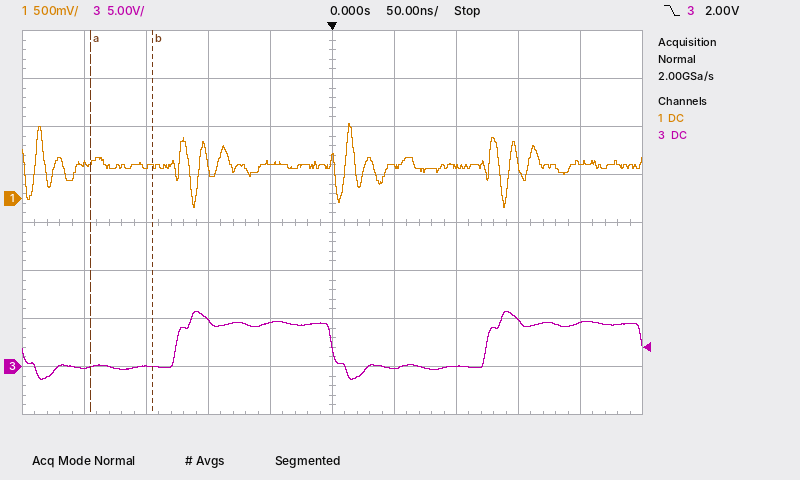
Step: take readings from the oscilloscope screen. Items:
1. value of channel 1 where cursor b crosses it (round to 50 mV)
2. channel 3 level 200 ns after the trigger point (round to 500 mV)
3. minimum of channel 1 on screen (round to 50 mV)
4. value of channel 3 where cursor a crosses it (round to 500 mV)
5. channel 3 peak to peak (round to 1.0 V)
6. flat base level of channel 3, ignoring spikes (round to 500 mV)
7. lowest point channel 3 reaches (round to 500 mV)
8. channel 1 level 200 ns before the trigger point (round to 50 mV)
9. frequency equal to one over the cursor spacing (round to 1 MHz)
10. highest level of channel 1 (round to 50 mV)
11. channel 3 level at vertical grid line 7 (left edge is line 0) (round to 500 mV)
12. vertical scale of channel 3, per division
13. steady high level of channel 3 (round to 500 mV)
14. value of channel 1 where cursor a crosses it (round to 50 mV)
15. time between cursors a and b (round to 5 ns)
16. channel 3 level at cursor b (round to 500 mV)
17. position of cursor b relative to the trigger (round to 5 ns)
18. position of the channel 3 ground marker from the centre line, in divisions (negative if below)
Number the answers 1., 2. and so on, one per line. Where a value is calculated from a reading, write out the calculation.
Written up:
1. 350 mV
2. 4.5 V
3. -100 mV
4. 0.0 V
5. 7.0 V
6. 0.0 V
7. -1.5 V
8. 350 mV
9. 1 / 50 ns ≈ 20 MHz
10. 800 mV
11. 0.0 V
12. 5 V
13. 4.5 V
14. 350 mV
15. 50 ns
16. 0.0 V
17. -145 ns
18. -3.0 div
